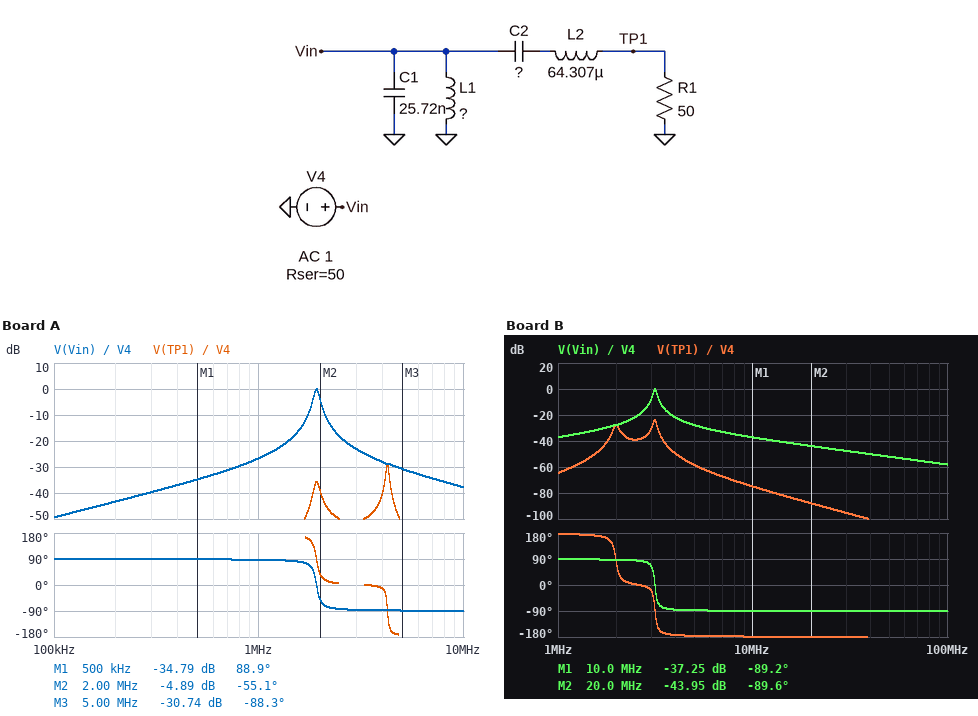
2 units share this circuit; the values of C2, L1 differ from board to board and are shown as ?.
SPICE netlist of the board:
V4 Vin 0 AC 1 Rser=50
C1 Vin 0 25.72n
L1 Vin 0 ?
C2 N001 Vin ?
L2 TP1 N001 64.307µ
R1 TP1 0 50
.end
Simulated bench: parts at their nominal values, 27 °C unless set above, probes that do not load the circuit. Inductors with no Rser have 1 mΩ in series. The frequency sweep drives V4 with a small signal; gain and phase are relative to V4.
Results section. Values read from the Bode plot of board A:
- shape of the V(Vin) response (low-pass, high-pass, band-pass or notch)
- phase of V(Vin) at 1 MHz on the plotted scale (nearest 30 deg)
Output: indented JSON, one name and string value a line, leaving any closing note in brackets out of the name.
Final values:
{
  "shape of the V(Vin) response": "band-pass",
  "phase of V(Vin) at 1 MHz on the plotted scale": "90 deg"
}
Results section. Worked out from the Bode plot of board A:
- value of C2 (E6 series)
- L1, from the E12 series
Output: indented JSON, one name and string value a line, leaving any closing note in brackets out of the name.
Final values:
{
  "value of C2": "22 pF",
  "L1, from the E12 series": "270 nH"
}
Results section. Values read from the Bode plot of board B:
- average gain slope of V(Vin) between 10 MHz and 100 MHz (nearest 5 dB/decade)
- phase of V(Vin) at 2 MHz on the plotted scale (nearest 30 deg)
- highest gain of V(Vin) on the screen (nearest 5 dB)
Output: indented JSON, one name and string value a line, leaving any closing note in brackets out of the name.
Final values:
{
  "average gain slope of V(Vin) between 10 MHz and 100 MHz": "-20 dB/decade",
  "phase of V(Vin) at 2 MHz on the plotted scale": "90 deg",
  "highest gain of V(Vin) on the screen": "0 dB"
}
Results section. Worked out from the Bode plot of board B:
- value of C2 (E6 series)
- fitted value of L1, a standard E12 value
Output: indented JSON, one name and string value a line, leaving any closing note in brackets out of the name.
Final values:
{
  "value of C2": "100 pF",
  "fitted value of L1, a standard E12 value": "100 nH"
}
